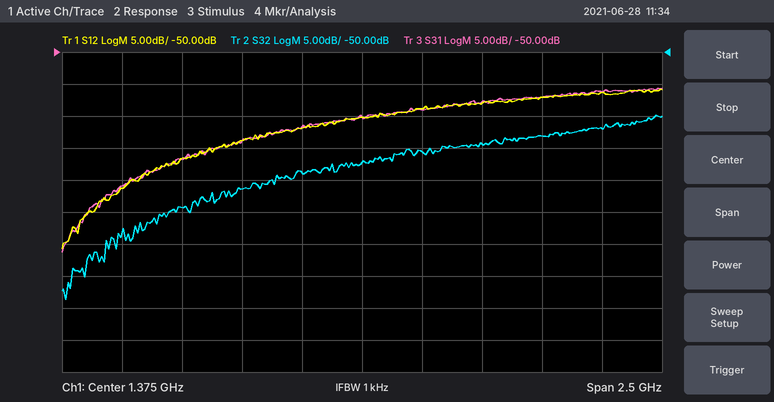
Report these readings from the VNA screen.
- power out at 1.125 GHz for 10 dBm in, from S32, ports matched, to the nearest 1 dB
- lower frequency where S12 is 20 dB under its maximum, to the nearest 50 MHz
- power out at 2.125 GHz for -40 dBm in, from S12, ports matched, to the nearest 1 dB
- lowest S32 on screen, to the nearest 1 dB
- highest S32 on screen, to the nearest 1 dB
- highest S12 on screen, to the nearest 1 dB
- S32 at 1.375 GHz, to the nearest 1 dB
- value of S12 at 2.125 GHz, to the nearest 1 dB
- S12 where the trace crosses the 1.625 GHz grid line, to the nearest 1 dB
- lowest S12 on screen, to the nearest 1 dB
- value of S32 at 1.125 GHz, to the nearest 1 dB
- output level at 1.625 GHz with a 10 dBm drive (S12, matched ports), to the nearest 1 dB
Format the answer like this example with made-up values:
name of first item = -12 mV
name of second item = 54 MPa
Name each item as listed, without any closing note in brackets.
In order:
power out at 1.125 GHz for 10 dBm in, from S32, ports matched, to the nearest 1 dB = -59 dBm
lower frequency where S12 is 20 dB under its maximum, to the nearest 50 MHz = 200 MHz
power out at 2.125 GHz for -40 dBm in, from S12, ports matched, to the nearest 1 dB = -97 dBm
lowest S32 on screen, to the nearest 1 dB = -89 dB
highest S32 on screen, to the nearest 1 dB = -60 dB
highest S12 on screen, to the nearest 1 dB = -56 dB
S32 at 1.375 GHz, to the nearest 1 dB = -67 dB
value of S12 at 2.125 GHz, to the nearest 1 dB = -57 dB
S12 where the trace crosses the 1.625 GHz grid line, to the nearest 1 dB = -59 dB
lowest S12 on screen, to the nearest 1 dB = -81 dB
value of S32 at 1.125 GHz, to the nearest 1 dB = -69 dB
output level at 1.625 GHz with a 10 dBm drive (S12, matched ports), to the nearest 1 dB = -49 dBm
